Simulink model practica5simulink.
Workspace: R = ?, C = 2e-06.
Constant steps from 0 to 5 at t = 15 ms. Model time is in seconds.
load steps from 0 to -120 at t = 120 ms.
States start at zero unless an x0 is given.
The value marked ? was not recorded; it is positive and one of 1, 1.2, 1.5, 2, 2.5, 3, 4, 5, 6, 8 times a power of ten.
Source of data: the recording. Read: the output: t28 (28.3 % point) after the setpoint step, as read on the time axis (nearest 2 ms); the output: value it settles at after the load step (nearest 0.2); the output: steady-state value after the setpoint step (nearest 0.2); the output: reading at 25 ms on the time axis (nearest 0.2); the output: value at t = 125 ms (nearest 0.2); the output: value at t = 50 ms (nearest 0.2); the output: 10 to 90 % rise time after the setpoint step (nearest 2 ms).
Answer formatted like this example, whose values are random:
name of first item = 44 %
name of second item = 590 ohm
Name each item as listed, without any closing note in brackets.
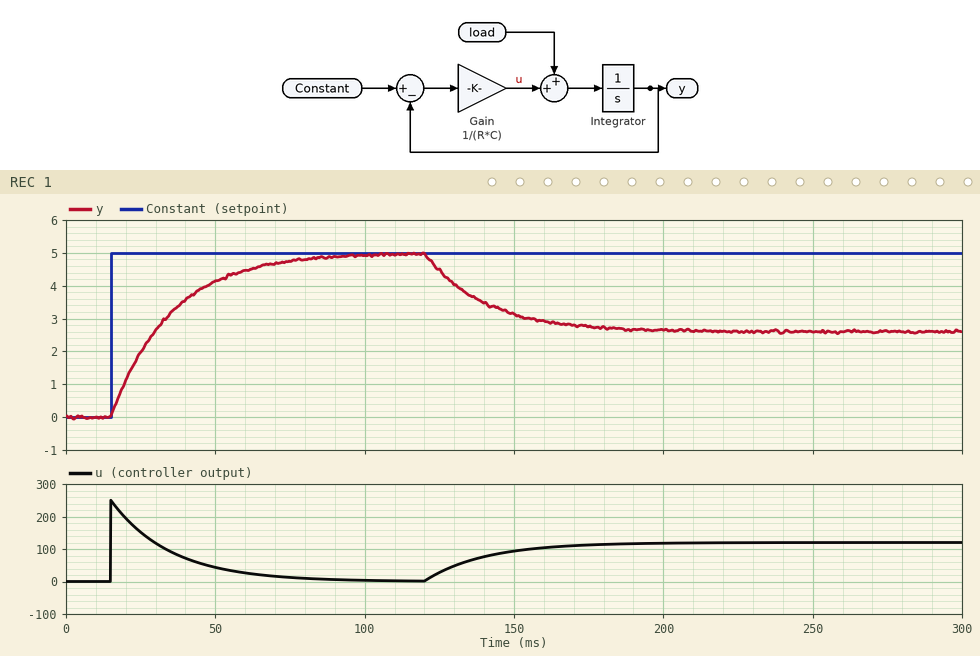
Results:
the output: t28 (28.3 % point) after the setpoint step, as read on the time axis = 22 ms
the output: value it settles at after the load step = 2.6
the output: steady-state value after the setpoint step = 5.0
the output: reading at 25 ms on the time axis = 2.0
the output: value at t = 125 ms = 4.4
the output: value at t = 50 ms = 4.2
the output: 10 to 90 % rise time after the setpoint step = 44 ms
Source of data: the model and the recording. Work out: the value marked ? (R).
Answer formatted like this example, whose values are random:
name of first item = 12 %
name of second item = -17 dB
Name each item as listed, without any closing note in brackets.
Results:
the value marked ? = 10000
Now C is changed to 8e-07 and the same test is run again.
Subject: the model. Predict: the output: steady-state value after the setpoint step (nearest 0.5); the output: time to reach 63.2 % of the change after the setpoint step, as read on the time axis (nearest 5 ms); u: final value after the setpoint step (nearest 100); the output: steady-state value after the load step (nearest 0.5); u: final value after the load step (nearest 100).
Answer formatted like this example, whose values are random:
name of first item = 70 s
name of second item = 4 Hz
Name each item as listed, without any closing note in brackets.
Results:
the output: steady-state value after the setpoint step = 5.0
the output: time to reach 63.2 % of the change after the setpoint step, as read on the time axis = 25 ms
u: final value after the setpoint step = 0
the output: steady-state value after the load step = 4.0
u: final value after the load step = 100
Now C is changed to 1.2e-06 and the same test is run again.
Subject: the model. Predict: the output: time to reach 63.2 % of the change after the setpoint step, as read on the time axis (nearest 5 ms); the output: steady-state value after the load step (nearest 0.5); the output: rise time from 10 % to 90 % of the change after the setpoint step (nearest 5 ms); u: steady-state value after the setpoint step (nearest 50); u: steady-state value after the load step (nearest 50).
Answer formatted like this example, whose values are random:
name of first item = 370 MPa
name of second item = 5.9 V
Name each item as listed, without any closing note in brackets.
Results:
the output: time to reach 63.2 % of the change after the setpoint step, as read on the time axis = 25 ms
the output: steady-state value after the load step = 3.5
the output: rise time from 10 % to 90 % of the change after the setpoint step = 25 ms
u: steady-state value after the setpoint step = 0
u: steady-state value after the load step = 100
